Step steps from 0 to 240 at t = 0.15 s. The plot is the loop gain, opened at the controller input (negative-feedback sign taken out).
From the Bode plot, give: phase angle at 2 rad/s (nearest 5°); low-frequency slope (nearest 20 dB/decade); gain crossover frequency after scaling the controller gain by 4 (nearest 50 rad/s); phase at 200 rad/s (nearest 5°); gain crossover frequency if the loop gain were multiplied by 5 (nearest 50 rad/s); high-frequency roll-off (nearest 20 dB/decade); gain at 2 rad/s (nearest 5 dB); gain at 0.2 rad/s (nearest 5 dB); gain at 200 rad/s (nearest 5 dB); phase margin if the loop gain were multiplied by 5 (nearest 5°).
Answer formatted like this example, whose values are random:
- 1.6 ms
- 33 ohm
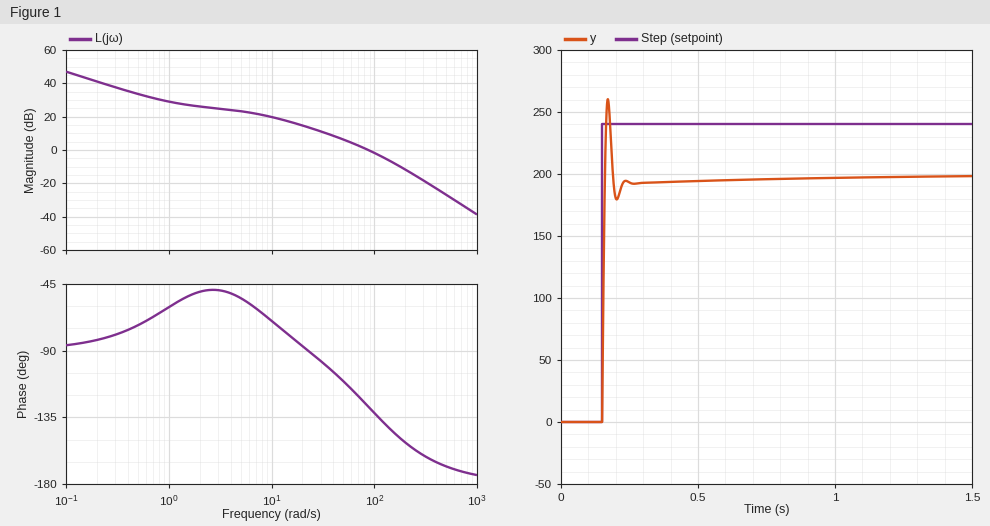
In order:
- -50°
- -20 dB/decade
- 200 rad/s
- -150°
- 250 rad/s
- -40 dB/decade
- 25 dB
- 40 dB
- -10 dB
- 25°
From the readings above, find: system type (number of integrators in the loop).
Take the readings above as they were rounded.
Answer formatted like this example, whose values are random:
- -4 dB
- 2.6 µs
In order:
- 1
